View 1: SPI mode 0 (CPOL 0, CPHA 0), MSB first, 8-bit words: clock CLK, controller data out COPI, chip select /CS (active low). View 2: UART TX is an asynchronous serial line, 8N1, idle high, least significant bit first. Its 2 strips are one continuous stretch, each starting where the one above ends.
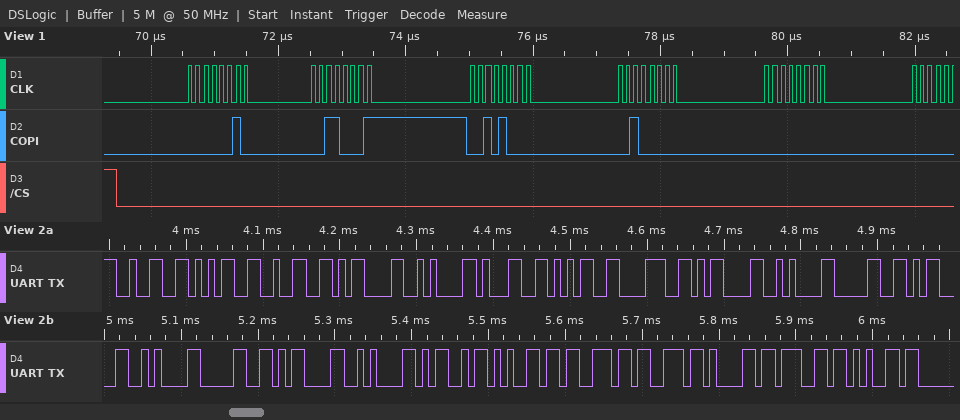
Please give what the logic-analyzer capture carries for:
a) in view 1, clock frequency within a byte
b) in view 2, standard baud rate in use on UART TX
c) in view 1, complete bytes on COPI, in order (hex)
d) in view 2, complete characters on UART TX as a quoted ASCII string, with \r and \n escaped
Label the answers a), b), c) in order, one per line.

a) 8 MHz
b) 115200 baud
c) 02 31 28 20 00
d) "252\r\n158\r\n0\r\n0\r\nMessage"
